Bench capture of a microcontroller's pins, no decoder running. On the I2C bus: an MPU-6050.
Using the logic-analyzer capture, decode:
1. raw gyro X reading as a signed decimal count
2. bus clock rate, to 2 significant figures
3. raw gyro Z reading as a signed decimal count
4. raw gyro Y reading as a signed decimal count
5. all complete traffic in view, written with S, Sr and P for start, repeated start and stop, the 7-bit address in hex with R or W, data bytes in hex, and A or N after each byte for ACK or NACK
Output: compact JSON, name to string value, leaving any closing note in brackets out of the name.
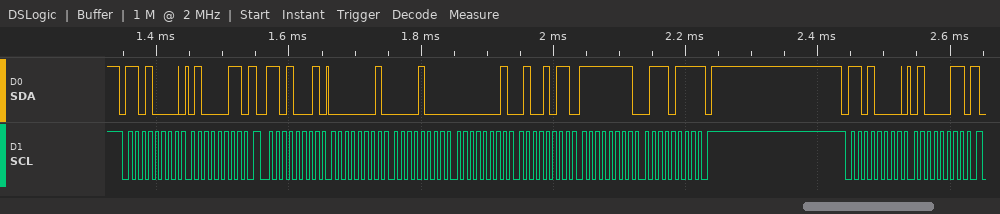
{"raw gyro X reading as a signed decimal count": "264", "bus clock rate, to 2 significant figures": "100 kHz", "raw gyro Z reading as a signed decimal count": "-137", "raw gyro Y reading as a signed decimal count": "331", "all complete traffic in view, written with S, Sr and P for start, repeated start and stop, the 7-bit address in hex with R or W, data bytes in hex, and A or N after each byte for ACK or NACK": "S 68W A 43 A Sr 68R A 01 A 08 A 01 A 4B A FF A 77 N P S 68W A 43 A"}
